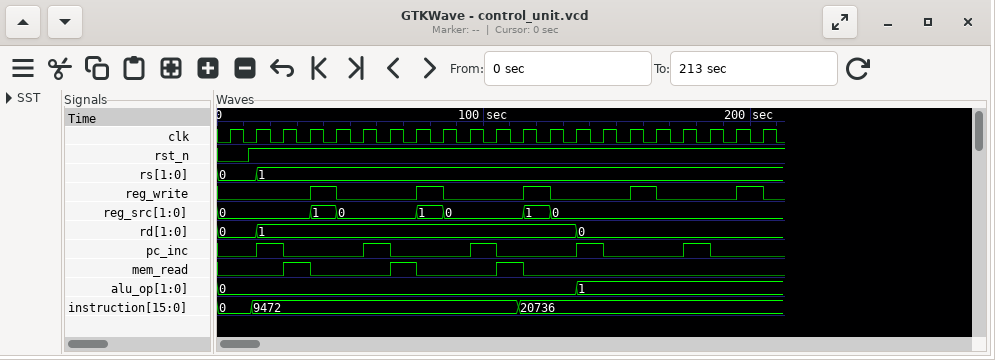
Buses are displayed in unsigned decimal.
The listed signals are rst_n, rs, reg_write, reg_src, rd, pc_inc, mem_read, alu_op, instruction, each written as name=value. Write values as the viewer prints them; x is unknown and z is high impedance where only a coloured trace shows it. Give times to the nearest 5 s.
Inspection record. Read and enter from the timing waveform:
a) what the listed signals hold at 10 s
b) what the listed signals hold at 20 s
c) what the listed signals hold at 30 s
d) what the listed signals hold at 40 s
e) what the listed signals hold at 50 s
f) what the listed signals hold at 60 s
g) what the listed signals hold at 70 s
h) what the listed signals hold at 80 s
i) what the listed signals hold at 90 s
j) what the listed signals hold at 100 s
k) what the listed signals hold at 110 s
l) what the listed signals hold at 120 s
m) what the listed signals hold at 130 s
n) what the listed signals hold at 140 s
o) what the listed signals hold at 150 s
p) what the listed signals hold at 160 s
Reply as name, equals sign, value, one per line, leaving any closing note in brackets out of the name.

what the listed signals hold at 10 s = rst_n=0, rs=0, reg_write=0, reg_src=0, rd=0, pc_inc=0, mem_read=0, alu_op=0, instruction=0
what the listed signals hold at 20 s = rst_n=1, rs=1, reg_write=0, reg_src=0, rd=1, pc_inc=1, mem_read=0, alu_op=0, instruction=9472
what the listed signals hold at 30 s = rst_n=1, rs=1, reg_write=0, reg_src=0, rd=1, pc_inc=0, mem_read=1, alu_op=0, instruction=9472
what the listed signals hold at 40 s = rst_n=1, rs=1, reg_write=1, reg_src=1, rd=1, pc_inc=0, mem_read=0, alu_op=0, instruction=9472
what the listed signals hold at 50 s = rst_n=1, rs=1, reg_write=0, reg_src=0, rd=1, pc_inc=0, mem_read=0, alu_op=0, instruction=9472
what the listed signals hold at 60 s = rst_n=1, rs=1, reg_write=0, reg_src=0, rd=1, pc_inc=1, mem_read=0, alu_op=0, instruction=9472
what the listed signals hold at 70 s = rst_n=1, rs=1, reg_write=0, reg_src=0, rd=1, pc_inc=0, mem_read=1, alu_op=0, instruction=9472
what the listed signals hold at 80 s = rst_n=1, rs=1, reg_write=1, reg_src=1, rd=1, pc_inc=0, mem_read=0, alu_op=0, instruction=9472
what the listed signals hold at 90 s = rst_n=1, rs=1, reg_write=0, reg_src=0, rd=1, pc_inc=0, mem_read=0, alu_op=0, instruction=9472
what the listed signals hold at 100 s = rst_n=1, rs=1, reg_write=0, reg_src=0, rd=1, pc_inc=1, mem_read=0, alu_op=0, instruction=9472
what the listed signals hold at 110 s = rst_n=1, rs=1, reg_write=0, reg_src=0, rd=1, pc_inc=0, mem_read=1, alu_op=0, instruction=9472
what the listed signals hold at 120 s = rst_n=1, rs=1, reg_write=1, reg_src=1, rd=1, pc_inc=0, mem_read=0, alu_op=0, instruction=20736
what the listed signals hold at 130 s = rst_n=1, rs=1, reg_write=0, reg_src=0, rd=1, pc_inc=0, mem_read=0, alu_op=0, instruction=20736
what the listed signals hold at 140 s = rst_n=1, rs=1, reg_write=0, reg_src=0, rd=0, pc_inc=1, mem_read=0, alu_op=1, instruction=20736
what the listed signals hold at 150 s = rst_n=1, rs=1, reg_write=0, reg_src=0, rd=0, pc_inc=0, mem_read=0, alu_op=1, instruction=20736
what the listed signals hold at 160 s = rst_n=1, rs=1, reg_write=1, reg_src=0, rd=0, pc_inc=0, mem_read=0, alu_op=1, instruction=20736
